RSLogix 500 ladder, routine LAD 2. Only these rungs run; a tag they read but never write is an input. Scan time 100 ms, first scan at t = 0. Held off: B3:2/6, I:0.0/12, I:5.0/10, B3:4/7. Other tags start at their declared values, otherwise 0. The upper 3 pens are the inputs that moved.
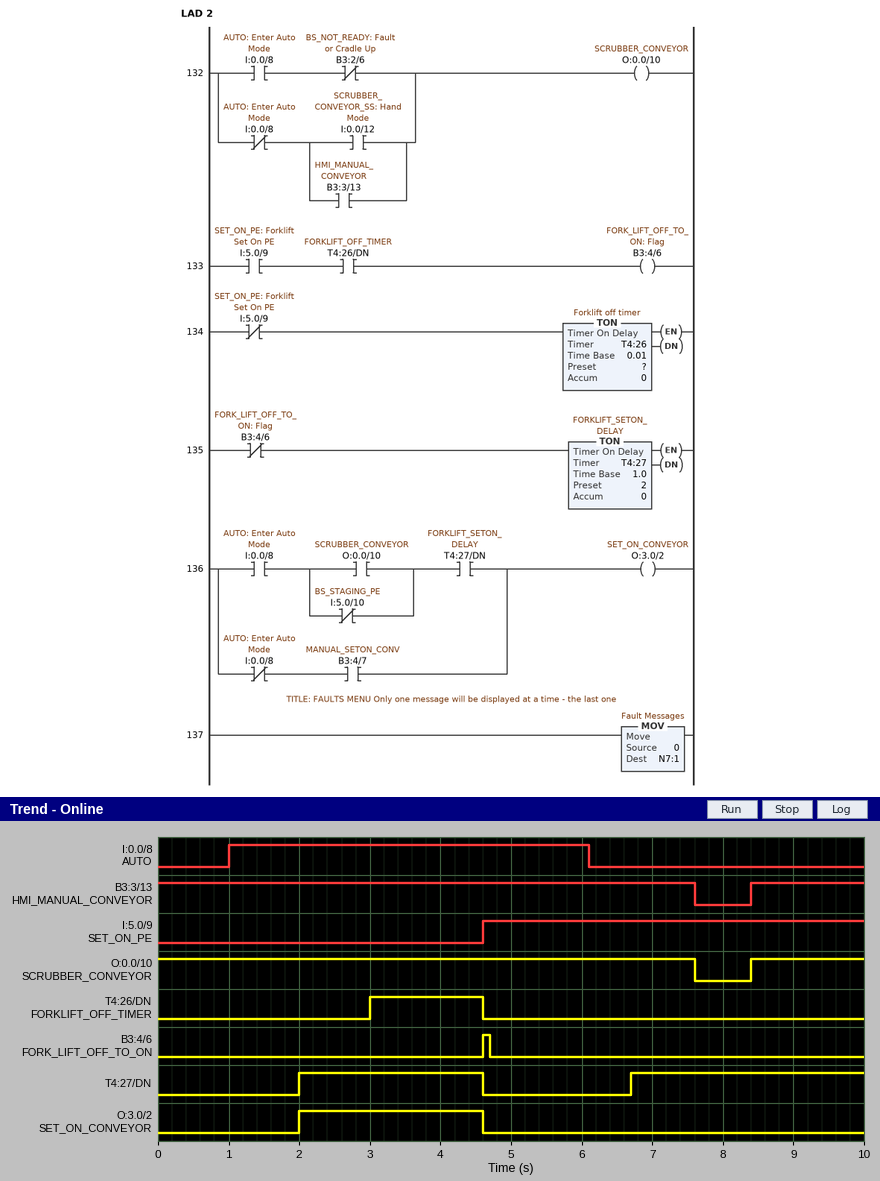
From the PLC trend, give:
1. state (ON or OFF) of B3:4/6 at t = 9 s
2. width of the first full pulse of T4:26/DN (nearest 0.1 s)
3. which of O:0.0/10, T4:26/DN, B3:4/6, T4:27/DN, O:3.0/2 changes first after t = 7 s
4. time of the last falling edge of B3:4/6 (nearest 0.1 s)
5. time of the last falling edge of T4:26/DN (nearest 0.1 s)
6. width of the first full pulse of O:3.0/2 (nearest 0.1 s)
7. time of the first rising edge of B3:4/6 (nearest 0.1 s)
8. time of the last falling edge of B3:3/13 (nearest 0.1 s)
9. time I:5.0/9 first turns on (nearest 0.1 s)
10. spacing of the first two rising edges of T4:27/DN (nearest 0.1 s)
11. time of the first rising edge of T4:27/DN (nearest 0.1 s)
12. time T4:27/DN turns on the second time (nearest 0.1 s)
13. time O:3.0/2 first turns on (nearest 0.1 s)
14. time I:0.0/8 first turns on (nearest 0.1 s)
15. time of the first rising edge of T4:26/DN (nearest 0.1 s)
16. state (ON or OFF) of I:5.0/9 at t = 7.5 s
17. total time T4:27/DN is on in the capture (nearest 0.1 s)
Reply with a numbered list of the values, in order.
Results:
1. OFF
2. 1.6 s
3. O:0.0/10
4. 4.7 s
5. 4.6 s
6. 2.6 s
7. 4.6 s
8. 7.6 s
9. 4.6 s
10. 4.7 s
11. 2.0 s
12. 6.7 s
13. 2.0 s
14. 1.0 s
15. 3.0 s
16. ON
17. 5.9 s
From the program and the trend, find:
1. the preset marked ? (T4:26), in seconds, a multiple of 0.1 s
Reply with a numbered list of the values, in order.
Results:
1. 3.0 s
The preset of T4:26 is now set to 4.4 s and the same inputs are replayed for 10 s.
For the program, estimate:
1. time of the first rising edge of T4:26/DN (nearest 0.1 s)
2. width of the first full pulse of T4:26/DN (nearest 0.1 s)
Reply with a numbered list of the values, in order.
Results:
1. 4.4 s
2. 0.2 s
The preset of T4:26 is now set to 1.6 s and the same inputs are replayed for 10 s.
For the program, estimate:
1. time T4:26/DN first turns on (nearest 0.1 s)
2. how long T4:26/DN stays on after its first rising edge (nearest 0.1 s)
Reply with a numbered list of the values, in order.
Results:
1. 1.6 s
2. 3.0 s
